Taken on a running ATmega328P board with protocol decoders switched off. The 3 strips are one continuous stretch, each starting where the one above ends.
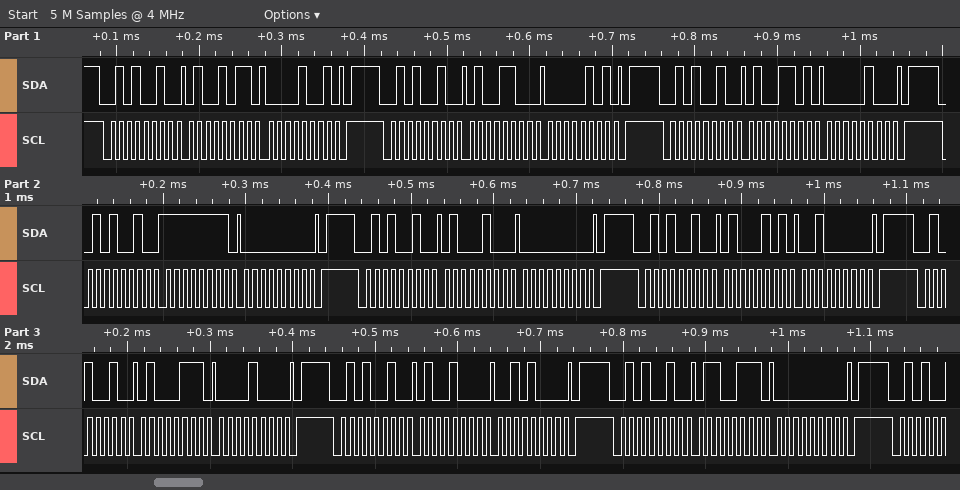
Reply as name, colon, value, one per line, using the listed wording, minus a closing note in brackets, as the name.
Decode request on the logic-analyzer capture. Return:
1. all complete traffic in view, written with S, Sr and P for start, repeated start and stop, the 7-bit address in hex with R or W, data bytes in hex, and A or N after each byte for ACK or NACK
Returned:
all complete traffic in view, written with S, Sr and P for start, repeated start and stop, the 7-bit address in hex with R or W, data bytes in hex, and A or N after each byte for ACK or NACK: S 29W A 4B A 09 A P S 29W A 4C A 05 A P S 29W A 4D A 04 A P S 29W A FF A 00 A P S 29W A 44 A 00 A P S 29W A 45 A 20 A P S 29W A 47 A 08 A P S 29W A 48 A 28 A P S 29W A 67 A 00 A P
